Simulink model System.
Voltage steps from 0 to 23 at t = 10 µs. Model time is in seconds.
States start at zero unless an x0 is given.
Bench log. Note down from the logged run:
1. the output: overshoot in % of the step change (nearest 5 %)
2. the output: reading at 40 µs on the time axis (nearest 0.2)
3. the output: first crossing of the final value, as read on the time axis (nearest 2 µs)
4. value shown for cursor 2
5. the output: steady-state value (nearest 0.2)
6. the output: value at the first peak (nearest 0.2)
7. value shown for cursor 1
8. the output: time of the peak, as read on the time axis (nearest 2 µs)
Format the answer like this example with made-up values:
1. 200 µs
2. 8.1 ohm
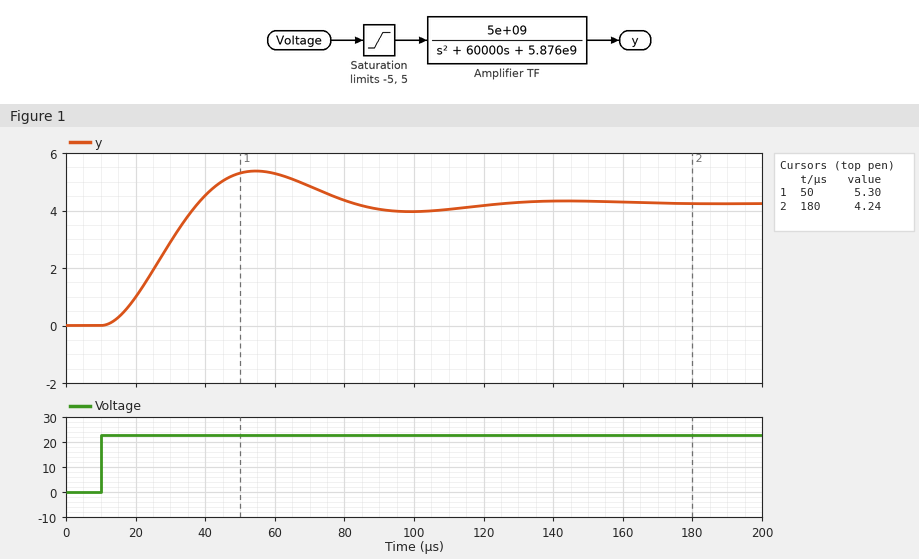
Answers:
1. 25 %
2. 4.6
3. 38 µs
4. 4.24
5. 4.2
6. 5.4
7. 5.30
8. 54 µs
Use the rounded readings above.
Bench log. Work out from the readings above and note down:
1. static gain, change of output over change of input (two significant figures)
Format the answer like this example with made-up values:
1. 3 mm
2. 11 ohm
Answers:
1. 0.18
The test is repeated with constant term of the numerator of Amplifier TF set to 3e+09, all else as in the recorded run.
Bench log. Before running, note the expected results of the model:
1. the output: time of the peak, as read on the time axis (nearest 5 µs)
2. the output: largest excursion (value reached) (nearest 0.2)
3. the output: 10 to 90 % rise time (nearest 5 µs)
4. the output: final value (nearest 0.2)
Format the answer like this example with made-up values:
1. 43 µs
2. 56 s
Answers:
1. 55 µs
2. 3.2
3. 20 µs
4. 2.6
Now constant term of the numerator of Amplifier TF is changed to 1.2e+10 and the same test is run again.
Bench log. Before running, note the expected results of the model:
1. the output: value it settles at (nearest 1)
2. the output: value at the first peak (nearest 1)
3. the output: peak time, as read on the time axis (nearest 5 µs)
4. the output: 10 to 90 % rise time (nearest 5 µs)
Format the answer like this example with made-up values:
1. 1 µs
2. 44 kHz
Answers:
1. 10
2. 13
3. 55 µs
4. 20 µs
